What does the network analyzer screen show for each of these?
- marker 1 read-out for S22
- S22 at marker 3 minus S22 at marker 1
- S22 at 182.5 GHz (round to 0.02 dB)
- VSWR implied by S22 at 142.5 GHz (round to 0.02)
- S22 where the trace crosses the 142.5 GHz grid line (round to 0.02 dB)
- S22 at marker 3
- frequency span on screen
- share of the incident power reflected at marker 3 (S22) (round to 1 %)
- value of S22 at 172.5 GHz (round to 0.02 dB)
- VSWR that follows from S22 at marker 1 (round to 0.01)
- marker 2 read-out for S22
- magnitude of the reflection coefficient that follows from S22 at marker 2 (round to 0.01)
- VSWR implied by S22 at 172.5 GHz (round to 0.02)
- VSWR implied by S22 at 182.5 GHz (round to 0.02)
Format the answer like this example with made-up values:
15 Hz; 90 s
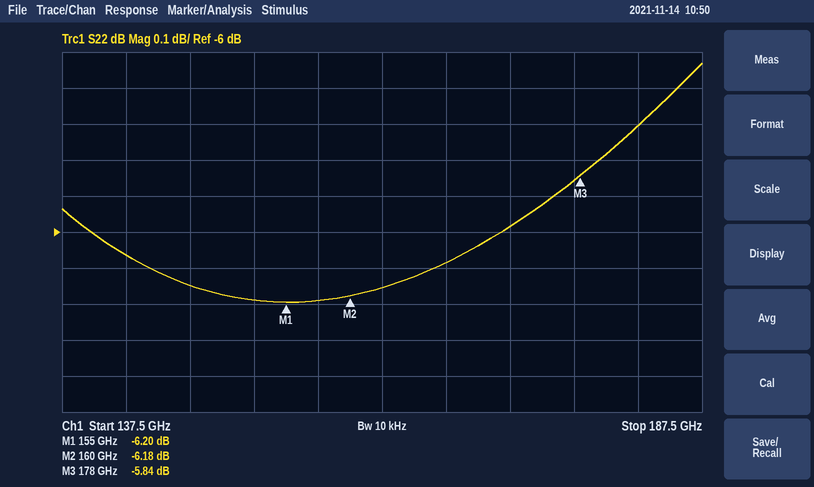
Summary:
-6.20 dB; 0.36 dB; -5.70 dB; 2.98; -6.06 dB; -5.84 dB; 50 GHz; 26 %; -5.98 dB; 2.92; -6.18 dB; 0.49; 3.02; 3.16
